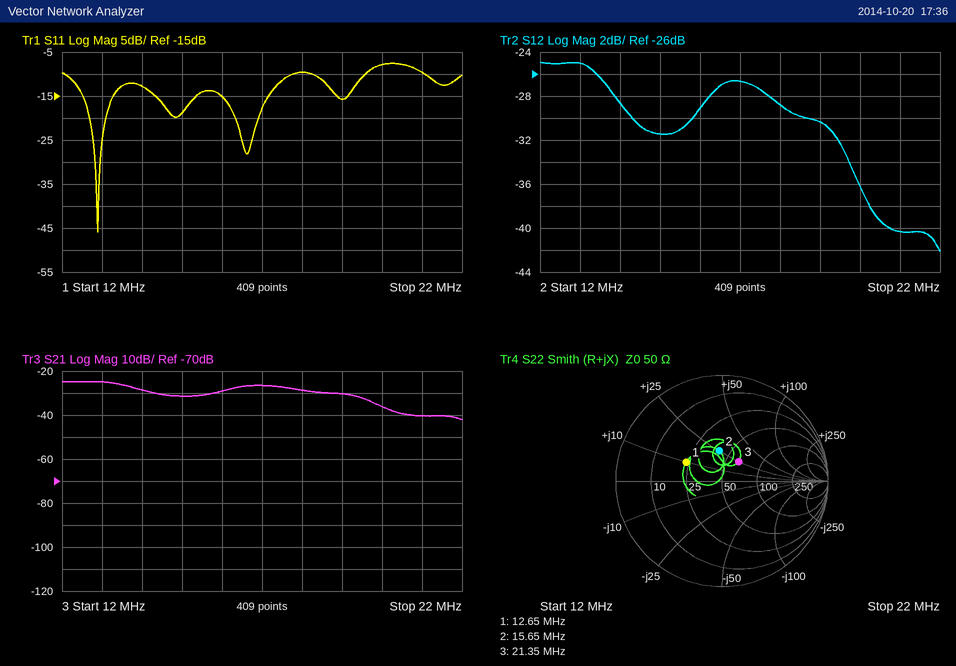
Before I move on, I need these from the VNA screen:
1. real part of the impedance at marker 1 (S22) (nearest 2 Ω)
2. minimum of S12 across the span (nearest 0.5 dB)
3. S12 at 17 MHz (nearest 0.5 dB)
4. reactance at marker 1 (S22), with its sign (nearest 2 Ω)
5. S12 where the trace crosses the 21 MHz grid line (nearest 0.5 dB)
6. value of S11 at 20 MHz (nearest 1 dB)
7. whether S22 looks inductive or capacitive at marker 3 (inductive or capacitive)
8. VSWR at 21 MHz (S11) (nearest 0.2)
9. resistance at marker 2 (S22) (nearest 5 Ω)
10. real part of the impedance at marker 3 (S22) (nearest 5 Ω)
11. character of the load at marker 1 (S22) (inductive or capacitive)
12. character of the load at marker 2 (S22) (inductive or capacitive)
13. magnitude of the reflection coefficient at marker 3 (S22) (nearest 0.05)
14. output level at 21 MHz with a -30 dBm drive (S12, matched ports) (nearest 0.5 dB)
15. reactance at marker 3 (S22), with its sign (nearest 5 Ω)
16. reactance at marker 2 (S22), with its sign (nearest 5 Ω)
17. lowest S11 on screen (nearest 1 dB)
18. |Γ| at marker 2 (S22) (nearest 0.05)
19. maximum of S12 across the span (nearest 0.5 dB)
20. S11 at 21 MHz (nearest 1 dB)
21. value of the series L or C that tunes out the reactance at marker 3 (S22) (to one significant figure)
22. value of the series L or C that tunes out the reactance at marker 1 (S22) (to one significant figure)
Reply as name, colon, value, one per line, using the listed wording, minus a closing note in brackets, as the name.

real part of the impedance at marker 1 (S22): 24 Ω
minimum of S12 across the span: -42.0 dB
S12 at 17 MHz: -26.5 dB
reactance at marker 1 (S22), with its sign: +10 Ω
S12 where the trace crosses the 21 MHz grid line: -40.5 dB
value of S11 at 20 MHz: -8 dB
whether S22 looks inductive or capacitive at marker 3: inductive
VSWR at 21 MHz (S11): 2.0
resistance at marker 2 (S22): 40 Ω
real part of the impedance at marker 3 (S22): 65 Ω
character of the load at marker 1 (S22): inductive
character of the load at marker 2 (S22): inductive
magnitude of the reflection coefficient at marker 3 (S22): 0.25
output level at 21 MHz with a -30 dBm drive (S12, matched ports): -70.5 dBm
reactance at marker 3 (S22), with its sign: +25 Ω
reactance at marker 2 (S22), with its sign: +25 Ω
lowest S11 on screen: -46 dB
|Γ| at marker 2 (S22): 0.30
maximum of S12 across the span: -25.0 dB
S11 at 21 MHz: -10 dB
value of the series L or C that tunes out the reactance at marker 3 (S22): 300 pF
value of the series L or C that tunes out the reactance at marker 1 (S22): 1 nF
